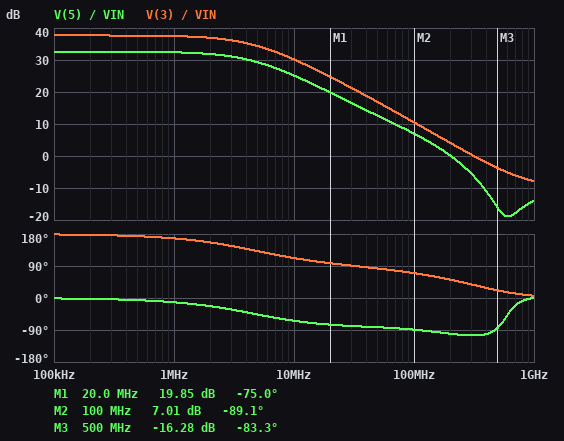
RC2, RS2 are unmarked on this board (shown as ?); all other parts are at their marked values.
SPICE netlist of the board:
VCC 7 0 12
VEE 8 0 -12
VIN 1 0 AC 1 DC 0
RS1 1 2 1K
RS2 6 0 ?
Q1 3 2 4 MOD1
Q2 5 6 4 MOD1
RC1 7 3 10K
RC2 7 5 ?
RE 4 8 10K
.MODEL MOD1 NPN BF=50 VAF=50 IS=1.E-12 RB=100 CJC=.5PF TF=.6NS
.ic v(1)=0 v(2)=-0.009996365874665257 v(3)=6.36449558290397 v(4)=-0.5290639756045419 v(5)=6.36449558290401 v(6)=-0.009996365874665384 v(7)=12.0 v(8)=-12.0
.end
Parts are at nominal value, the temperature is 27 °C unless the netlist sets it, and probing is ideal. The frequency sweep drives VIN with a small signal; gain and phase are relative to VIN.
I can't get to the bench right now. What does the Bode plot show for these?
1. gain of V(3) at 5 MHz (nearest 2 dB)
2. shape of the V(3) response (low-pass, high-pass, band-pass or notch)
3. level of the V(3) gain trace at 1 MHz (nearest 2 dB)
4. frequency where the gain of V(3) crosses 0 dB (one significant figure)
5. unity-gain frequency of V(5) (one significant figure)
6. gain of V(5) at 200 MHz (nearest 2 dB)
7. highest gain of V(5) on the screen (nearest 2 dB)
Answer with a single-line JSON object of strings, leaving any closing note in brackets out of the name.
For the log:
{"gain of V(3) at 5 MHz": "34 dB", "shape of the V(3) response": "low-pass", "level of the V(3) gain trace at 1 MHz": "38 dB", "frequency where the gain of V(3) crosses 0 dB": "300 MHz", "unity-gain frequency of V(5)": "200 MHz", "gain of V(5) at 200 MHz": "0 dB", "highest gain of V(5) on the screen": "32 dB"}
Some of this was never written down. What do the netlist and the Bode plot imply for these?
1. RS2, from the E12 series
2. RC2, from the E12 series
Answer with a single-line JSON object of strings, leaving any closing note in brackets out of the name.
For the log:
{"RS2, from the E12 series": "470 Ω", "RC2, from the E12 series": "5.6 kΩ"}
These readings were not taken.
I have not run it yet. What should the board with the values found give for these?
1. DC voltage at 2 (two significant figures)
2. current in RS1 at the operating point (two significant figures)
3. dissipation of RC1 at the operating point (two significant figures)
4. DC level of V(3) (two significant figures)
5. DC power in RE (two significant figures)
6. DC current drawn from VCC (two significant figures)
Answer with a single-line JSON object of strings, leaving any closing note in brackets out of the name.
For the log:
{"DC voltage at 2": "-9.0 mV", "current in RS1 at the operating point": "9.0 µA", "dissipation of RC1 at the operating point": "2.6 mW", "DC level of V(3)": "6.9 V", "DC power in RE": "13 mW", "DC current drawn from VCC": "1.1 mA"}
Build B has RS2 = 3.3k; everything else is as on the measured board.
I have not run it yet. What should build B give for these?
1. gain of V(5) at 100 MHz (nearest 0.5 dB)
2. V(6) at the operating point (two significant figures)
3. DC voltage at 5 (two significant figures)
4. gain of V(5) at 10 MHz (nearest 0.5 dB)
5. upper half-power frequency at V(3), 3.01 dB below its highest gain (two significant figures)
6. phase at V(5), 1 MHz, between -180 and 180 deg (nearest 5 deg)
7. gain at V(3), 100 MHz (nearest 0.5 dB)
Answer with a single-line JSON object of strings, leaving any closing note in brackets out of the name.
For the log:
{"gain of V(5) at 100 MHz": "-2.0 dB", "V(6) at the operating point": "-25 mV", "DC voltage at 5": "9.5 V", "gain of V(5) at 10 MHz": "19.0 dB", "upper half-power frequency at V(3), 3.01 dB below its highest gain": "3.0 MHz", "phase at V(5), 1 MHz, between -180 and 180 deg": "-20 deg", "gain at V(3), 100 MHz": "5.5 dB"}
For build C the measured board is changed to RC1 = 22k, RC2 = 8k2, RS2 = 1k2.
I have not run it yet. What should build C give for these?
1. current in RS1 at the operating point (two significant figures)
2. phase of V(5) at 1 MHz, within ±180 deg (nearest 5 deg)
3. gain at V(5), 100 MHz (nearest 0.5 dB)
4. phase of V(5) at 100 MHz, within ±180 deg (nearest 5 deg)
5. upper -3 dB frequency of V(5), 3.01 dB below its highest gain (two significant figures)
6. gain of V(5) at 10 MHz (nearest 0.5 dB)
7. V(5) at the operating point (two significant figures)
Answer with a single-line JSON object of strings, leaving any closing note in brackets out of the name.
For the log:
{"current in RS1 at the operating point": "11 µA", "phase of V(5) at 1 MHz, within ±180 deg": "-30 deg", "gain at V(5), 100 MHz": "4.5 dB", "phase of V(5) at 100 MHz, within ±180 deg": "-80 deg", "upper -3 dB frequency of V(5), 3.01 dB below its highest gain": "1.5 MHz", "gain of V(5) at 10 MHz": "19.0 dB", "V(5) at the operating point": "7.2 V"}
